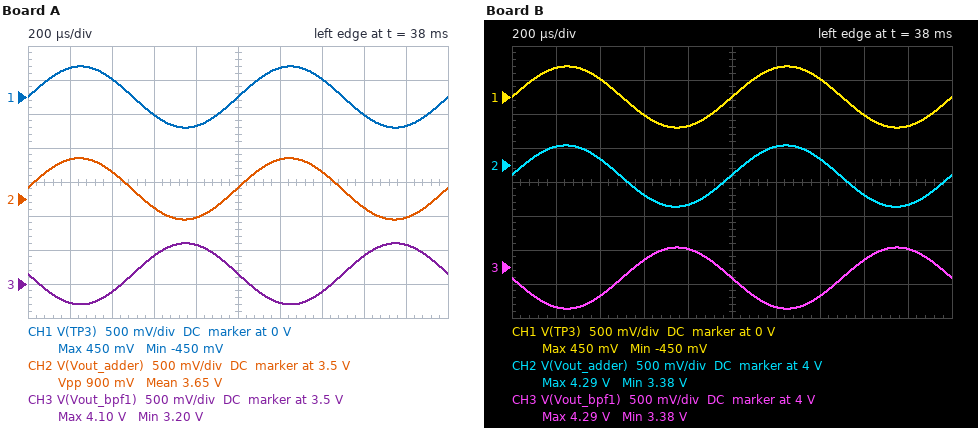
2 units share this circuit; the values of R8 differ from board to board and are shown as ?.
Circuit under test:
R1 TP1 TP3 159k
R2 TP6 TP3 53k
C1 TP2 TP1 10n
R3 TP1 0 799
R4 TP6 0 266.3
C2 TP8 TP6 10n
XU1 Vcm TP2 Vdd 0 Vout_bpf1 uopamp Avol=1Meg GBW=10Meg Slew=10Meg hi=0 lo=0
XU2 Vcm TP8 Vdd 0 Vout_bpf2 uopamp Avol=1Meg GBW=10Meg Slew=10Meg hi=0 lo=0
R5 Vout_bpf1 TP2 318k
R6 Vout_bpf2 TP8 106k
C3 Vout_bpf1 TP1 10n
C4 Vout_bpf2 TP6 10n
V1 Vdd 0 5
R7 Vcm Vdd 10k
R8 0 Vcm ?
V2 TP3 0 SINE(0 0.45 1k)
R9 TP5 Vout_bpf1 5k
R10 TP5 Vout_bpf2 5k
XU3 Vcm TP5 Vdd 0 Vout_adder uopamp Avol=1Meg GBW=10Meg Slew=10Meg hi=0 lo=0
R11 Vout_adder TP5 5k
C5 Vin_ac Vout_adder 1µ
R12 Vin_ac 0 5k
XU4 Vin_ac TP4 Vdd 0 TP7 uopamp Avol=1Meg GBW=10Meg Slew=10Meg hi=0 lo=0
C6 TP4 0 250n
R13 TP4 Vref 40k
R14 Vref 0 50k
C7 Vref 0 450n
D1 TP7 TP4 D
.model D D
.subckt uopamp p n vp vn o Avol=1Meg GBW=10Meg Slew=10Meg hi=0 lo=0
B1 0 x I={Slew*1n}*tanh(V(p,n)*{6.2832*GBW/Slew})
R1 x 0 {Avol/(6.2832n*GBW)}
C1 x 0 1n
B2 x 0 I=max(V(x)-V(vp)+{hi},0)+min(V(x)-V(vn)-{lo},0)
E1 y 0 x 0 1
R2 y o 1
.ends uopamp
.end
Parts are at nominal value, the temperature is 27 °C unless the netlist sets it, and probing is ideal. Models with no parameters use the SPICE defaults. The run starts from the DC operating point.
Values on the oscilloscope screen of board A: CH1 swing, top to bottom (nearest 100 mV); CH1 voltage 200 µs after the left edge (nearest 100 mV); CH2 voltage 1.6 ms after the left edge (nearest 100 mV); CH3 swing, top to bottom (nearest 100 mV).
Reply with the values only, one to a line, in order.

900 mV
400 mV
3.4 V
900 mV
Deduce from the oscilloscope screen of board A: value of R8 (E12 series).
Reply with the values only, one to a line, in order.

27 kΩ
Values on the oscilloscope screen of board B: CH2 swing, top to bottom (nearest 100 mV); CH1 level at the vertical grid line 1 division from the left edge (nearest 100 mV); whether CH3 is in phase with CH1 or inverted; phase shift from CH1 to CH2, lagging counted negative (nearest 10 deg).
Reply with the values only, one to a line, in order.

900 mV
400 mV
inverted
0 deg
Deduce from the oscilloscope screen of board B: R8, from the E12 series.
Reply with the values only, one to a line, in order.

33 kΩ
